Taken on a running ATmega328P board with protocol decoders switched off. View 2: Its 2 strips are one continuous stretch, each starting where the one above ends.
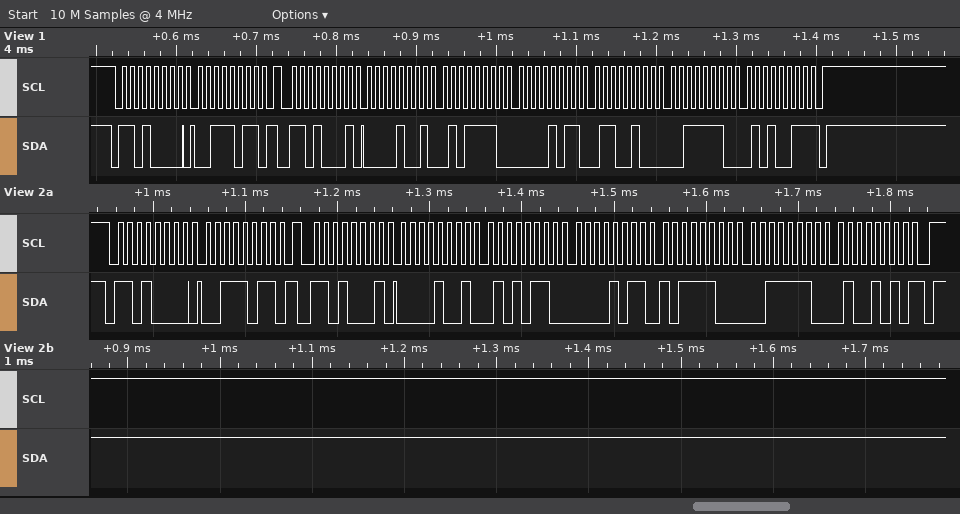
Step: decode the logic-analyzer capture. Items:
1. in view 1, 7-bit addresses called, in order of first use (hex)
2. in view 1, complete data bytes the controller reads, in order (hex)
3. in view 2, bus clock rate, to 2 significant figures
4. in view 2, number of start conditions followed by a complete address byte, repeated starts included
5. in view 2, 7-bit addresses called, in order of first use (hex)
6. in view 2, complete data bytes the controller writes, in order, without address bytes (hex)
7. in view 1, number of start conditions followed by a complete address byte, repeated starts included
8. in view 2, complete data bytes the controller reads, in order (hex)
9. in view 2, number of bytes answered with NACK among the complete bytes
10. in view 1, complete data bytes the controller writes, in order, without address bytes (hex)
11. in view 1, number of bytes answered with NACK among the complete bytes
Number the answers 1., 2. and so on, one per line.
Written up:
1. 0x68
2. 09 5E 0B 64 3E 53
3. 100 kHz
4. 2
5. 0x68
6. 3B
7. 2
8. 09 56 0B BC 3E 4A
9. 1
10. 3B
11. 1
